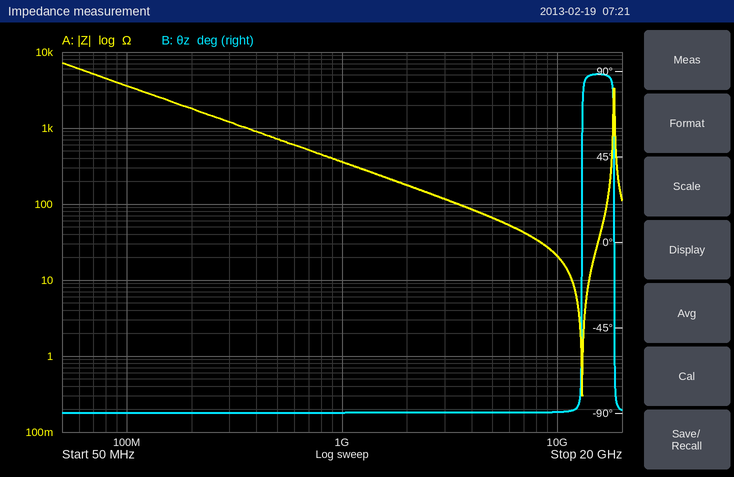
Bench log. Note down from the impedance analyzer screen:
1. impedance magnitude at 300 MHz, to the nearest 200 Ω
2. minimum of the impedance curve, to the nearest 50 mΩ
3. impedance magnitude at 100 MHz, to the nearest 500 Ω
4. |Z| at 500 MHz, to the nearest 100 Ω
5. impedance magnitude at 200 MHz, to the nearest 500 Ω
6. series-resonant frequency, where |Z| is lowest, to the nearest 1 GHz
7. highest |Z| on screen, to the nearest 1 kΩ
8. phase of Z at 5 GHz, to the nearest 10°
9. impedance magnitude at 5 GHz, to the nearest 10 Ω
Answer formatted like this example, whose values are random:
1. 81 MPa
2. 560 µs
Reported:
1. 1.2 kΩ
2. 300 mΩ
3. 3.5 kΩ
4. 700 Ω
5. 2.0 kΩ
6. 13 GHz
7. 7 kΩ
8. -90°
9. 70 Ω
